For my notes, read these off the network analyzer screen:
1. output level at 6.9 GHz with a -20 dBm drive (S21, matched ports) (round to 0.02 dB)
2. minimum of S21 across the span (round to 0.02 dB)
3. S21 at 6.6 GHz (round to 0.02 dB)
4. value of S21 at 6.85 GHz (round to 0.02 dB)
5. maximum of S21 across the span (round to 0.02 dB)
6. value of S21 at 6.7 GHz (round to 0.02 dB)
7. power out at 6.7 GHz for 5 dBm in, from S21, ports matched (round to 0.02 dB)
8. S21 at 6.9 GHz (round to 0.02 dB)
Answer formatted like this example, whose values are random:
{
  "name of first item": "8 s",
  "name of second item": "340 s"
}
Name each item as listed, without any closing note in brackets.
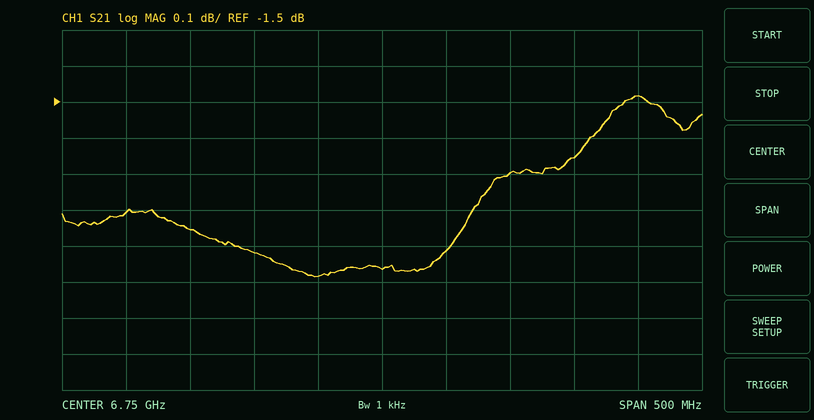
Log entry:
{
  "output level at 6.9 GHz with a -20 dBm drive (S21, matched ports)": "-21.66 dBm",
  "minimum of S21 across the span": "-1.98 dB",
  "S21 at 6.6 GHz": "-1.86 dB",
  "value of S21 at 6.85 GHz": "-1.70 dB",
  "maximum of S21 across the span": "-1.48 dB",
  "value of S21 at 6.7 GHz": "-1.98 dB",
  "power out at 6.7 GHz for 5 dBm in, from S21, ports matched": "3.02 dBm",
  "S21 at 6.9 GHz": "-1.66 dB"
}
